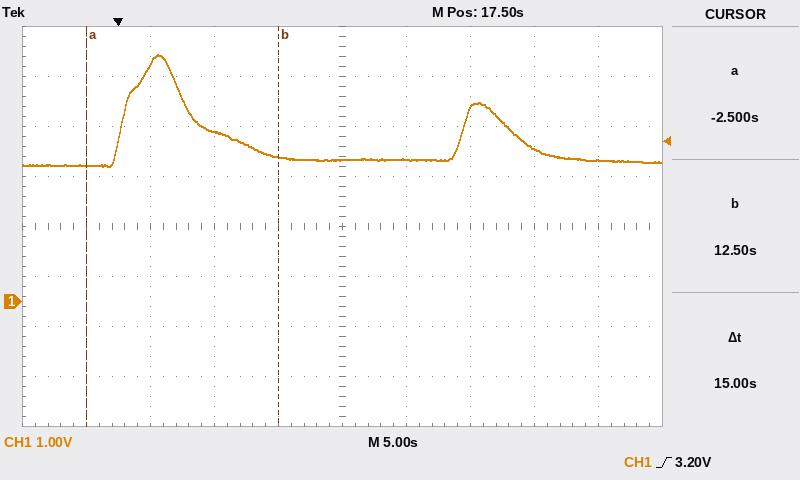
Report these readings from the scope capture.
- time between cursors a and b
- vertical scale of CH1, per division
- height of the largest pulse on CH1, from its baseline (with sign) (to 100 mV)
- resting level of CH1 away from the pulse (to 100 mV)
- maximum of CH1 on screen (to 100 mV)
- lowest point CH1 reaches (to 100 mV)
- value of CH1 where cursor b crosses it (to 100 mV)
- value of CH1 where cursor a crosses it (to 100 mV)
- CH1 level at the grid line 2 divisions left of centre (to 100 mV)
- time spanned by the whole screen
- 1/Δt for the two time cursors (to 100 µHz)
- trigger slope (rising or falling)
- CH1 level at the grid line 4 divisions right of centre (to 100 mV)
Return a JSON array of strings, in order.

["15 s", "1 V", "+2.1 V", "2.8 V", "4.9 V", "2.7 V", "2.9 V", "2.7 V", "3.4 V", "50 s", "66.7 mHz", "rising", "2.8 V"]
